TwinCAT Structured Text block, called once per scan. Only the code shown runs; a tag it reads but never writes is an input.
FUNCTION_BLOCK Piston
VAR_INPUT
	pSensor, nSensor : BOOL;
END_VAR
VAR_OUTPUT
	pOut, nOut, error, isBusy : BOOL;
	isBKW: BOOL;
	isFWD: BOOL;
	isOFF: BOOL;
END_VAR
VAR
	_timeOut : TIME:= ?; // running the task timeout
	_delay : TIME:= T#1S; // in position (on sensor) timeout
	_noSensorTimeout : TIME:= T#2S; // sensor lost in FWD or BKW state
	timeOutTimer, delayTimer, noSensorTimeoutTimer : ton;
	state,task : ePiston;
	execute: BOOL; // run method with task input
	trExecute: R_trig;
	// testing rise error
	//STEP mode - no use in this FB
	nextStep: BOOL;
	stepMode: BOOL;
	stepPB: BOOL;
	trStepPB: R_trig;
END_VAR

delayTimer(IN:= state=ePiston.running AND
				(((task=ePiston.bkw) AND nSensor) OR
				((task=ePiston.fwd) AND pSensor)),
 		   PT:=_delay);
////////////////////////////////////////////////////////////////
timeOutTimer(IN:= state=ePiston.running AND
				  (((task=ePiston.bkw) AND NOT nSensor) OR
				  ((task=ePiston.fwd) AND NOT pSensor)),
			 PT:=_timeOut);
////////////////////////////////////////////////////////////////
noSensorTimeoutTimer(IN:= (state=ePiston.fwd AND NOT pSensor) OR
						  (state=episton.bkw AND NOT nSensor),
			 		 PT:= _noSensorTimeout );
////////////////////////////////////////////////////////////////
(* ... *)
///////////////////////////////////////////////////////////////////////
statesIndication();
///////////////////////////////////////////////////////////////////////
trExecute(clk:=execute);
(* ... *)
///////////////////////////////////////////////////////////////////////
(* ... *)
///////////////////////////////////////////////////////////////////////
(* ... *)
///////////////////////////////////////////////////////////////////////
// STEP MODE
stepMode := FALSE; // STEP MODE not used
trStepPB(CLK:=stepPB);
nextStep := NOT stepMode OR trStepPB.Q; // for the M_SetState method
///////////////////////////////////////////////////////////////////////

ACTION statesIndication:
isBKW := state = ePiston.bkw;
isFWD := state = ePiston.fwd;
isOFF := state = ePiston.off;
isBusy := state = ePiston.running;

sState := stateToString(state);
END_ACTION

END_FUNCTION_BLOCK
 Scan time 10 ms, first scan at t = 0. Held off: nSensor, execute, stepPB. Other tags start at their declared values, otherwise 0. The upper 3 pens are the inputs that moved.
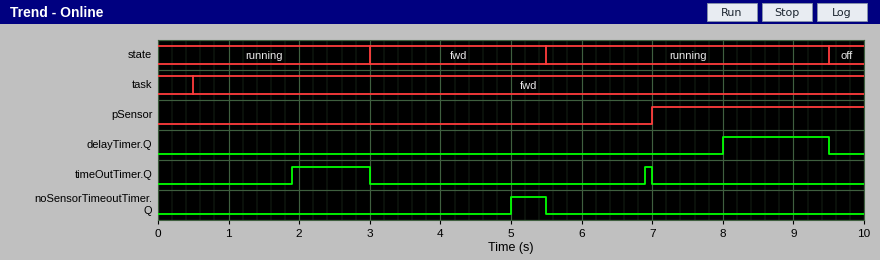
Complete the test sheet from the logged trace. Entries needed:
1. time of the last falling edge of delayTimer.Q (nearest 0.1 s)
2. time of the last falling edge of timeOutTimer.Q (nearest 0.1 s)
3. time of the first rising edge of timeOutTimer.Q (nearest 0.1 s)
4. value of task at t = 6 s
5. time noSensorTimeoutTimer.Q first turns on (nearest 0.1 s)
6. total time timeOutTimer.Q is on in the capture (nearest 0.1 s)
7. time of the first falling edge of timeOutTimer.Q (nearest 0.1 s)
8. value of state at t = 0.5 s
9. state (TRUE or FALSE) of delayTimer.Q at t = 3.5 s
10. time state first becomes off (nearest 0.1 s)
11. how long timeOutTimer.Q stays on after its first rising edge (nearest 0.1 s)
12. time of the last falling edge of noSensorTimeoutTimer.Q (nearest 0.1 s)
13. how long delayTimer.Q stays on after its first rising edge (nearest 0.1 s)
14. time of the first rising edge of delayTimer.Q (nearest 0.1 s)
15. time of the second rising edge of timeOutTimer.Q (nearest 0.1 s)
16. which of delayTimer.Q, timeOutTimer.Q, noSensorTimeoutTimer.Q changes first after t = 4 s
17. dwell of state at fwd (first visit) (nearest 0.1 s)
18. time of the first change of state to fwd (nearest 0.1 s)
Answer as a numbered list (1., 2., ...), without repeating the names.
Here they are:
1. 9.5 s
2. 7.0 s
3. 1.9 s
4. fwd
5. 5.0 s
6. 1.2 s
7. 3.0 s
8. running
9. FALSE
10. 9.5 s
11. 1.1 s
12. 5.5 s
13. 1.5 s
14. 8.0 s
15. 6.9 s
16. noSensorTimeoutTimer.Q
17. 2.5 s
18. 3.0 s
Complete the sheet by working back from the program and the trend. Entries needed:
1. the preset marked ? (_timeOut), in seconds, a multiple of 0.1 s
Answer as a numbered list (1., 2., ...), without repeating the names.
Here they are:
1. 1.4 s
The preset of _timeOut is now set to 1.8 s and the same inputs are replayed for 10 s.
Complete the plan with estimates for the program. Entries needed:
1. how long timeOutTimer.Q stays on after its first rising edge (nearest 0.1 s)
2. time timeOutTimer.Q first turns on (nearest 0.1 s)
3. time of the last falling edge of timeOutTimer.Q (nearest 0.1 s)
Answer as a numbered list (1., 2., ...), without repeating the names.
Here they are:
1. 0.7 s
2. 2.3 s
3. 3.0 s
